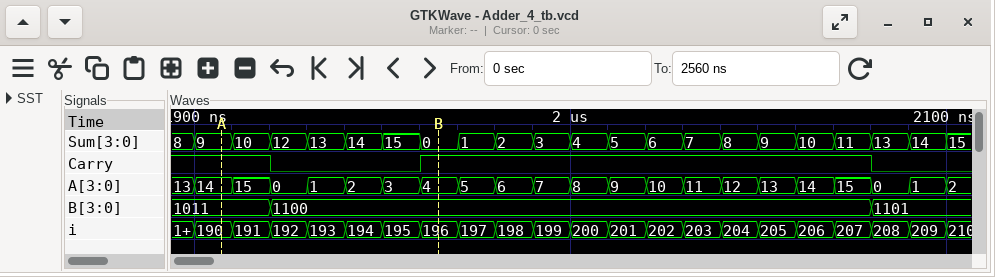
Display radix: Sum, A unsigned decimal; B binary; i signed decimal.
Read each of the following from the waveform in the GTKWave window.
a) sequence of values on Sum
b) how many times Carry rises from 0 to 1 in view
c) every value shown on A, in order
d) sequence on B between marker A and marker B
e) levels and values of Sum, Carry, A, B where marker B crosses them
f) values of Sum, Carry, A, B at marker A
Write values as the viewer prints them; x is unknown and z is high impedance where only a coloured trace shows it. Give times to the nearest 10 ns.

8, 9, 10, 12, 13, 14, 15, 0, 1, 2, 3, 4, 5, 6, 7, 8, 9, 10, 11, 13, 14, 15
1
13, 14, 15, 0, 1, 2, 3, 4, 5, 6, 7, 8, 9, 10, 11, 12, 13, 14, 15, 0, 1, 2
1011, 1100
Sum=0, Carry=1, A=4, B=1100
Sum=9, Carry=1, A=14, B=1011
